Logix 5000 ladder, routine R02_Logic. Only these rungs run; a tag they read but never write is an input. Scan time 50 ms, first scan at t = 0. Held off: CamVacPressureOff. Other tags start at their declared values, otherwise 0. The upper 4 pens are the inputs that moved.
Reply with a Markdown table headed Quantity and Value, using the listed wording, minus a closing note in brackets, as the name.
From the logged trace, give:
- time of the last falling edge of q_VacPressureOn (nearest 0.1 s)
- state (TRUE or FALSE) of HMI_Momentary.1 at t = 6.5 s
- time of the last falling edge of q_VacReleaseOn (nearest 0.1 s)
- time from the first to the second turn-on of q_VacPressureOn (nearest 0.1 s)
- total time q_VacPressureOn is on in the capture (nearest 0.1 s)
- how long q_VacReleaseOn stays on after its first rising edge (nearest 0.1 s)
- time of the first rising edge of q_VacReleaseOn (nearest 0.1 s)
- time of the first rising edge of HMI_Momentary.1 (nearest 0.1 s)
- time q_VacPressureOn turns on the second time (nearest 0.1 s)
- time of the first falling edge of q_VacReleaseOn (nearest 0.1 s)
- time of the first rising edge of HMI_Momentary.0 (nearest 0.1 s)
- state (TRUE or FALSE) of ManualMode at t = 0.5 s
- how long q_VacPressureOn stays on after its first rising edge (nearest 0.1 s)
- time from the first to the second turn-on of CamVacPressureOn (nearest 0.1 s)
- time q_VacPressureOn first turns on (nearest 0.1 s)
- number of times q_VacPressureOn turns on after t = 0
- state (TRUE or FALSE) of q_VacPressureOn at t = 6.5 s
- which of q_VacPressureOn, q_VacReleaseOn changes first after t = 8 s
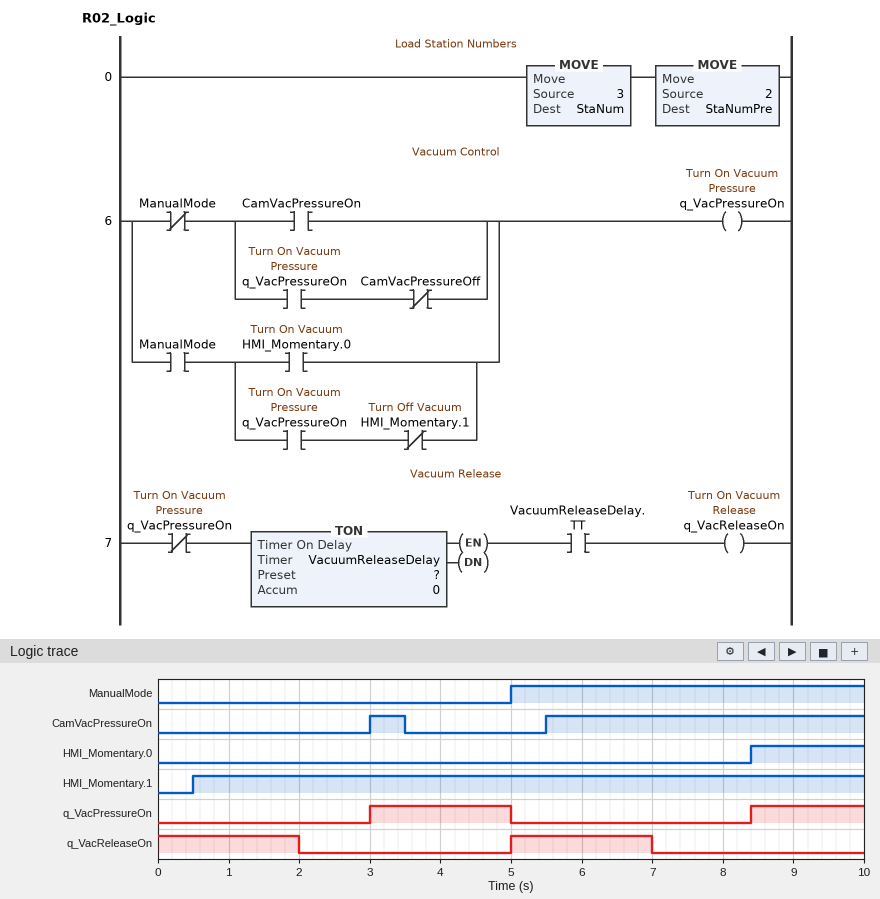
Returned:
| Quantity | Value |
|---|---|
| time of the last falling edge of q_VacPressureOn | 5.0 s |
| state (TRUE or FALSE) of HMI_Momentary.1 at t = 6.5 s | TRUE |
| time of the last falling edge of q_VacReleaseOn | 7.0 s |
| time from the first to the second turn-on of q_VacPressureOn | 5.4 s |
| total time q_VacPressureOn is on in the capture | 3.6 s |
| how long q_VacReleaseOn stays on after its first rising edge | 2.0 s |
| time of the first rising edge of q_VacReleaseOn | 5.0 s |
| time of the first rising edge of HMI_Momentary.1 | 0.5 s |
| time q_VacPressureOn turns on the second time | 8.4 s |
| time of the first falling edge of q_VacReleaseOn | 2.0 s |
| time of the first rising edge of HMI_Momentary.0 | 8.4 s |
| state (TRUE or FALSE) of ManualMode at t = 0.5 s | FALSE |
| how long q_VacPressureOn stays on after its first rising edge | 2.0 s |
| time from the first to the second turn-on of CamVacPressureOn | 2.5 s |
| time q_VacPressureOn first turns on | 3.0 s |
| number of times q_VacPressureOn turns on after t = 0 | 2 |
| state (TRUE or FALSE) of q_VacPressureOn at t = 6.5 s | FALSE |
| which of q_VacPressureOn, q_VacReleaseOn changes first after t = 8 s | q_VacPressureOn |
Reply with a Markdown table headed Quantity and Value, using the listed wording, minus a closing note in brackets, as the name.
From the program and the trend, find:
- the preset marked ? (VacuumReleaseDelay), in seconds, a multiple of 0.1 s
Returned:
| Quantity | Value |
|---|---|
| the preset marked ? (VacuumReleaseDelay), in seconds, a multiple of 0.1 s | 2.0 s |
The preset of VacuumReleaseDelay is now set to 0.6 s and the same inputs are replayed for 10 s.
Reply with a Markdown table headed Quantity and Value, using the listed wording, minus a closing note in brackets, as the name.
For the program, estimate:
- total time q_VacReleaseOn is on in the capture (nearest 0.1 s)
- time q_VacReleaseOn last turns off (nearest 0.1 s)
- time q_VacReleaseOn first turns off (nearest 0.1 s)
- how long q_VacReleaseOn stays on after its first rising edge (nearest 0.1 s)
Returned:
| Quantity | Value |
|---|---|
| total time q_VacReleaseOn is on in the capture | 1.2 s |
| time q_VacReleaseOn last turns off | 5.6 s |
| time q_VacReleaseOn first turns off | 0.6 s |
| how long q_VacReleaseOn stays on after its first rising edge | 0.6 s |
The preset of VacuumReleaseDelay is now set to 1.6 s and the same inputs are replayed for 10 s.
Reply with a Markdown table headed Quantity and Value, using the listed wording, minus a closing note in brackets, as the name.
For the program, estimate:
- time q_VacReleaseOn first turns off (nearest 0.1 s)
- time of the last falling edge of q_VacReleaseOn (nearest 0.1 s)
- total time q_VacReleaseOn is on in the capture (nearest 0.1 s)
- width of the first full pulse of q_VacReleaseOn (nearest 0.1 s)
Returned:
| Quantity | Value |
|---|---|
| time q_VacReleaseOn first turns off | 1.6 s |
| time of the last falling edge of q_VacReleaseOn | 6.6 s |
| total time q_VacReleaseOn is on in the capture | 3.2 s |
| width of the first full pulse of q_VacReleaseOn | 1.6 s |
